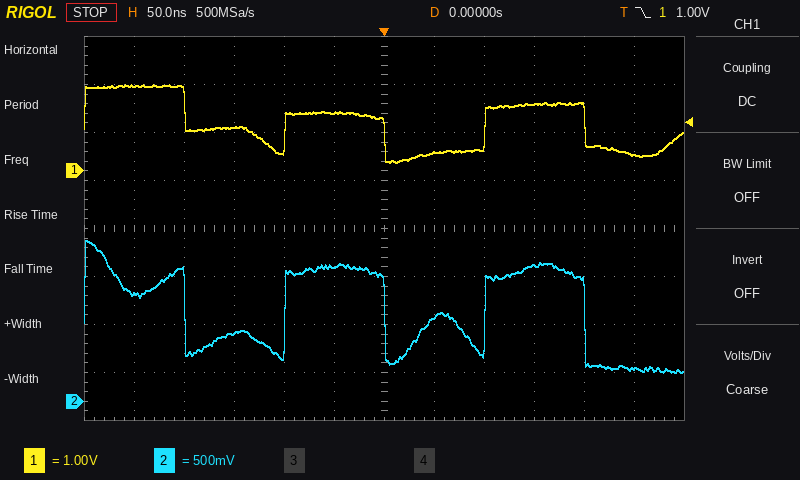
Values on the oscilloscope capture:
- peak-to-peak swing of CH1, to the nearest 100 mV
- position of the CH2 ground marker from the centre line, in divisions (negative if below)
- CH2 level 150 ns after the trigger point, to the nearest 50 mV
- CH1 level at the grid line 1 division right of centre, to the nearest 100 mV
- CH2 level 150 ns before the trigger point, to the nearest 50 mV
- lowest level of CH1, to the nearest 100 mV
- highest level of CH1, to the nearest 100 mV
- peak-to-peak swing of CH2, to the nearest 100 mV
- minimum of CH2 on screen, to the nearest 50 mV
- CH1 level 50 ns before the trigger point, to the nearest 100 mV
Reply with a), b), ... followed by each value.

a) 1.6 V
b) -3.6 div
c) 1.40 V
d) 400 mV
e) 700 mV
f) 200 mV
g) 1.8 V
h) 1.40 V
i) 300 mV
j) 1.2 V
